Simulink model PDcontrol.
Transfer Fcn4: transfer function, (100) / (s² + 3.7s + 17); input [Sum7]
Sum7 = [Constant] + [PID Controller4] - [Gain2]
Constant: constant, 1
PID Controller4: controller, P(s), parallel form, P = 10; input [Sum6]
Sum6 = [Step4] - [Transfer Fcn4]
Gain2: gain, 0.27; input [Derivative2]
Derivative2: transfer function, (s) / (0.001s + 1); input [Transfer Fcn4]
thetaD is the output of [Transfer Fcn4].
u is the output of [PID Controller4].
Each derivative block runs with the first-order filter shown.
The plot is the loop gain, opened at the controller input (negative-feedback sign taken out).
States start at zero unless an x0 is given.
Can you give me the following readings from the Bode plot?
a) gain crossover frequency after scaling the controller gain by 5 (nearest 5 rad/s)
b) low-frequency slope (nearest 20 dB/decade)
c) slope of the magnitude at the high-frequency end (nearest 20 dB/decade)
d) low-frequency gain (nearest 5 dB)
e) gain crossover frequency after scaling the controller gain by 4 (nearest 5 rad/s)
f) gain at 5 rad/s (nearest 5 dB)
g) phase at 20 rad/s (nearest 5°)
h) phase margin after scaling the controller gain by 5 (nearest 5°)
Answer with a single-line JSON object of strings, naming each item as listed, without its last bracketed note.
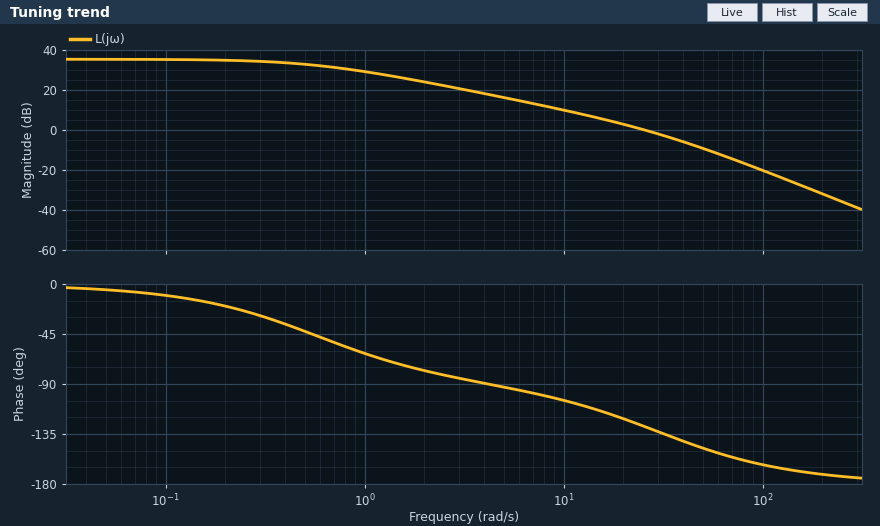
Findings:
{"gain crossover frequency after scaling the controller gain by 5": "70 rad/s", "low-frequency slope": "0 dB/decade", "slope of the magnitude at the high-frequency end": "-40 dB/decade", "low-frequency gain": "35 dB", "gain crossover frequency after scaling the controller gain by 4": "60 rad/s", "gain at 5 rad/s": "15 dB", "phase at 20 rad/s": "-120°", "phase margin after scaling the controller gain by 5": "25°"}
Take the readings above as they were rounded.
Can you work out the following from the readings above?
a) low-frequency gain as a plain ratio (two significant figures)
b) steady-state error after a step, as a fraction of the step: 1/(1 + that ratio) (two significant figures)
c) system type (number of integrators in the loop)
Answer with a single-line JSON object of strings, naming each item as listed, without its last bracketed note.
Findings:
{"low-frequency gain as a plain ratio": "56", "steady-state error after a step, as a fraction of the step: 1/(1 + that ratio)": "0.018", "system type": "0"}
